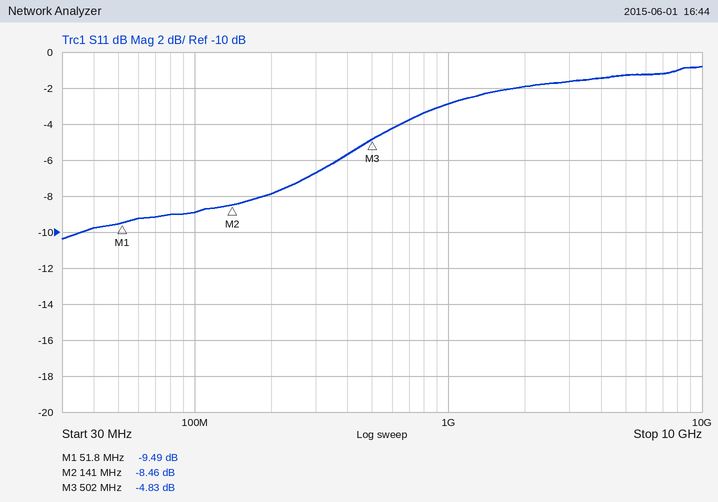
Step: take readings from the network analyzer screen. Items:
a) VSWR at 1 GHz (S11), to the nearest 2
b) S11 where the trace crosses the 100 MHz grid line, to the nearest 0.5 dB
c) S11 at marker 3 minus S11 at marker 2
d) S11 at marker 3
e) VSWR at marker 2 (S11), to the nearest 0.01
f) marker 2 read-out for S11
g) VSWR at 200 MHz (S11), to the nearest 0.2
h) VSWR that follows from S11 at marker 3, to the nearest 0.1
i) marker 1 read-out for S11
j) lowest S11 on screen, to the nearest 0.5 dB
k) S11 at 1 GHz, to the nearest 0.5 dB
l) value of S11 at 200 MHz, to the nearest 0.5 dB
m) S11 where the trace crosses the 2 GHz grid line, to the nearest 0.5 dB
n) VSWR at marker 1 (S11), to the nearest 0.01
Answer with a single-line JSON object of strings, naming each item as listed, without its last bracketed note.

{"VSWR at 1 GHz (S11), to the nearest 2": "6", "S11 where the trace crosses the 100 MHz grid line, to the nearest 0.5 dB": "-9.0 dB", "S11 at marker 3 minus S11 at marker 2": "3.63 dB", "S11 at marker 3": "-4.83 dB", "VSWR at marker 2 (S11), to the nearest 0.01": "2.21", "marker 2 read-out for S11": "-8.46 dB", "VSWR at 200 MHz (S11), to the nearest 0.2": "2.4", "VSWR that follows from S11 at marker 3, to the nearest 0.1": "3.7", "marker 1 read-out for S11": "-9.49 dB", "lowest S11 on screen, to the nearest 0.5 dB": "-10.5 dB", "S11 at 1 GHz, to the nearest 0.5 dB": "-3.0 dB", "value of S11 at 200 MHz, to the nearest 0.5 dB": "-8.0 dB", "S11 where the trace crosses the 2 GHz grid line, to the nearest 0.5 dB": "-2.0 dB", "VSWR at marker 1 (S11), to the nearest 0.01": "2.01"}
